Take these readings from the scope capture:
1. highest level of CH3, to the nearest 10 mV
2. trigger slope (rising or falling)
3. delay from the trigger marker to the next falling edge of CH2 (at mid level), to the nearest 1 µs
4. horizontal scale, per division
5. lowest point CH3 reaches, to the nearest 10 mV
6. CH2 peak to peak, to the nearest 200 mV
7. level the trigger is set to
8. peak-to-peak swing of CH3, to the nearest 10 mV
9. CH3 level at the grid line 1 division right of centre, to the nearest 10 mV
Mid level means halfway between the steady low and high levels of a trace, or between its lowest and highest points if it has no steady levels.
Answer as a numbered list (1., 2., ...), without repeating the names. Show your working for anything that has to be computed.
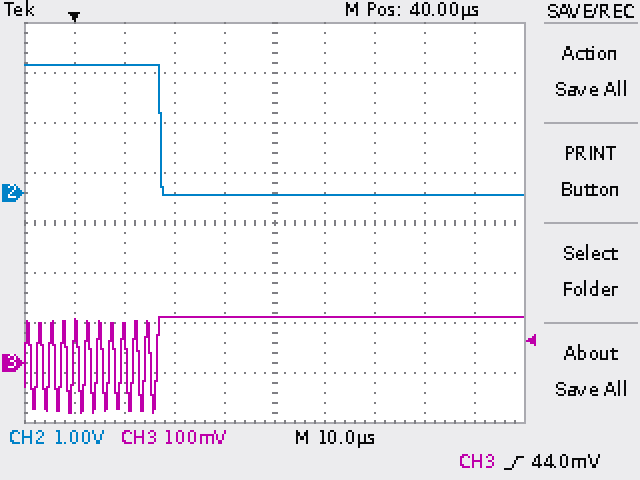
1. 90 mV
2. rising
3. 17 µs
4. 10 µs
5. -100 mV
6. 2.6 V
7. 44.0 mV
8. 90 mV − (-100 mV) = 190 mV
9. 90 mV
